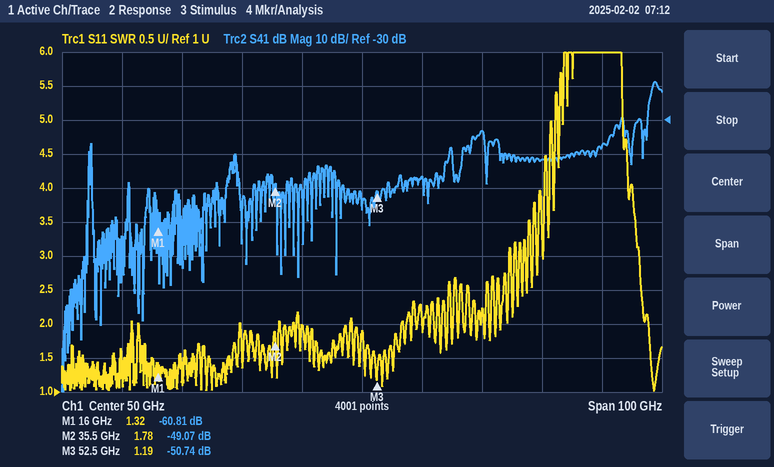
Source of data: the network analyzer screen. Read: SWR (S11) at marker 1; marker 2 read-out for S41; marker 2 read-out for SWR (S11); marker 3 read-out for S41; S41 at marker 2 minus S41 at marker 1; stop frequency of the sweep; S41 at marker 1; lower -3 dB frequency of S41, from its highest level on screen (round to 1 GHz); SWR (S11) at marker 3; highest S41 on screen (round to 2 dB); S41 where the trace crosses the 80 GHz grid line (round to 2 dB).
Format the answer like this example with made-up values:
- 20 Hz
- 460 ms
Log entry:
- 1.32
- -49.07 dB
- 1.78
- -50.74 dB
- 11.74 dB
- 100 GHz
- -60.81 dB
- 98 GHz
- 1.19
- -18 dB
- -42 dB
